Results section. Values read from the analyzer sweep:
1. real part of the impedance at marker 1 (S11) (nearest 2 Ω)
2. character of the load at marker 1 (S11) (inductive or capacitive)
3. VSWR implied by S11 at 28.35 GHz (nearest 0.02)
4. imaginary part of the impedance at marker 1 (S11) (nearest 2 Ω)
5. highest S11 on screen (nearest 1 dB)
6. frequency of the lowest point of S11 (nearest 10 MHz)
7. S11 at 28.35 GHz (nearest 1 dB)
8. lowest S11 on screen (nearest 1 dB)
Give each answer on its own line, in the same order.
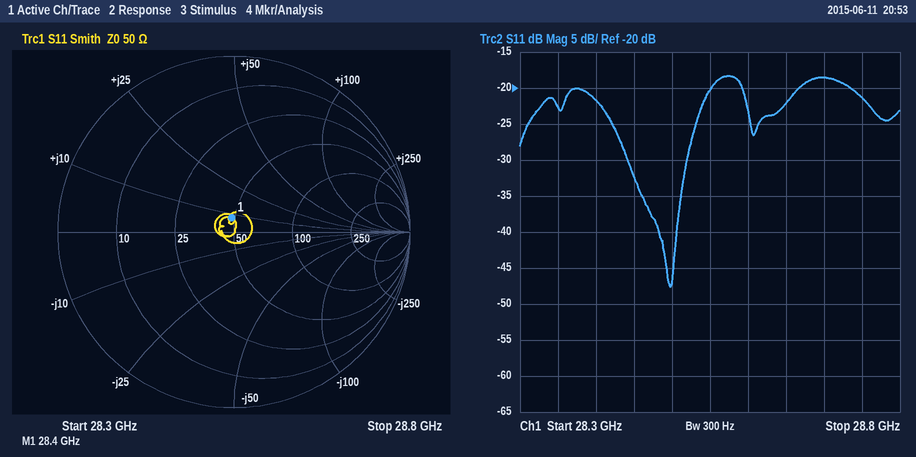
48 Ω
inductive
1.16
+8 Ω
-18 dB
28.50 GHz
-23 dB
-48 dB
